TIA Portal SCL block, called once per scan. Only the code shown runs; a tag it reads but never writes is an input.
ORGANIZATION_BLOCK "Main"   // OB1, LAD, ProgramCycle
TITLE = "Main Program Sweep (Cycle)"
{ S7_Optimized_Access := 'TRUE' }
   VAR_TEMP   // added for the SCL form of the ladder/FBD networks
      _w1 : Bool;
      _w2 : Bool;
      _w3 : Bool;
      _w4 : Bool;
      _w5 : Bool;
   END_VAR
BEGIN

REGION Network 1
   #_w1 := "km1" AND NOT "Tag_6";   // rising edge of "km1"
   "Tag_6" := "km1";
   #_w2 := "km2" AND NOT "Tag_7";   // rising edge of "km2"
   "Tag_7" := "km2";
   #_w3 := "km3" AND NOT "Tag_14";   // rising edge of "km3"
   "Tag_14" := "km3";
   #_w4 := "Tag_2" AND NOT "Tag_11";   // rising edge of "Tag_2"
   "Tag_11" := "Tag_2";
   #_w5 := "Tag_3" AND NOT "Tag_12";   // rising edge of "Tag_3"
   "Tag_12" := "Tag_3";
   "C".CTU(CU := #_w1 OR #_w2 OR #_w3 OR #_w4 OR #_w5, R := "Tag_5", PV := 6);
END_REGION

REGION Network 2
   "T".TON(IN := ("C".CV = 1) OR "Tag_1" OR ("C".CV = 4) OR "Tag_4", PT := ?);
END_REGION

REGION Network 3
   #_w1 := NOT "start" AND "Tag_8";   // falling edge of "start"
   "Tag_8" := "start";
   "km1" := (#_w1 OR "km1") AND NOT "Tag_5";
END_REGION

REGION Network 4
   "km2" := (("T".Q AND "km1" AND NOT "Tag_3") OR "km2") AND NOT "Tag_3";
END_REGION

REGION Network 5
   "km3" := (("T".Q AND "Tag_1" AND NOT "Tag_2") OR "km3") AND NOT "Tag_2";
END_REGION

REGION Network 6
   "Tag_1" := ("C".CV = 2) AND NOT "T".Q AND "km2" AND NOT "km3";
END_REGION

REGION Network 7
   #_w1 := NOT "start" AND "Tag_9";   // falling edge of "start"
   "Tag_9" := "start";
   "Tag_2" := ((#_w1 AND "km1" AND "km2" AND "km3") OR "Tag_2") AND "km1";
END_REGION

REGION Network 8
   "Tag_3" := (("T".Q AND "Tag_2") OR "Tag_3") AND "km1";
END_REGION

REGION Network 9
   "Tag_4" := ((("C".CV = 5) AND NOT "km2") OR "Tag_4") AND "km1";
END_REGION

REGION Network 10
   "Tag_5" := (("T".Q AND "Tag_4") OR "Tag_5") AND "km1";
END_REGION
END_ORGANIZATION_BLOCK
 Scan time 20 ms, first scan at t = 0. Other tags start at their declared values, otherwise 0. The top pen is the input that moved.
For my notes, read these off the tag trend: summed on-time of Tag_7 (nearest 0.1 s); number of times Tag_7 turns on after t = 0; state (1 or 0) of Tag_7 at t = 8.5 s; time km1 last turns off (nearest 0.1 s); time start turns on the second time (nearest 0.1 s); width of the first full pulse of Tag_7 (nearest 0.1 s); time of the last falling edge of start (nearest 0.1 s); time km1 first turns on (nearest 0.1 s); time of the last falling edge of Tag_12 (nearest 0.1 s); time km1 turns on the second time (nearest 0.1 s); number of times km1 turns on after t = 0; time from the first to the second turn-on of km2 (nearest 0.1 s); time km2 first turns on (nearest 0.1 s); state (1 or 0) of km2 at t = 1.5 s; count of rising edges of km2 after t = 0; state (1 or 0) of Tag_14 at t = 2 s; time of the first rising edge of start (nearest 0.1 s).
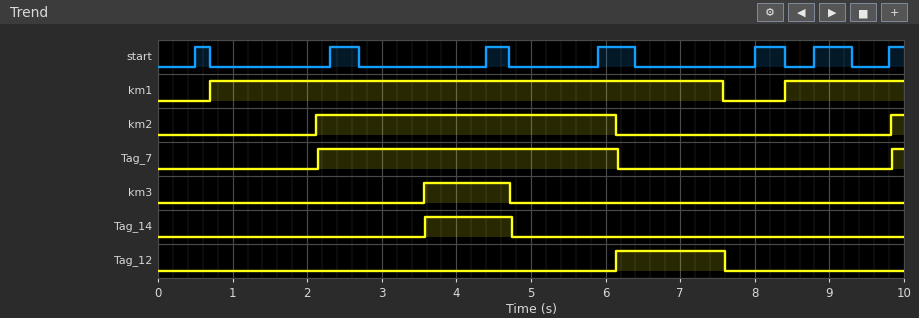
4.2 s
2
0
7.6 s
2.3 s
4.0 s
9.3 s
0.7 s
7.6 s
8.4 s
2
7.7 s
2.1 s
0
2
0
0.5 s
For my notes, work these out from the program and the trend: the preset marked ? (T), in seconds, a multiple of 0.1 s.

1.4 s
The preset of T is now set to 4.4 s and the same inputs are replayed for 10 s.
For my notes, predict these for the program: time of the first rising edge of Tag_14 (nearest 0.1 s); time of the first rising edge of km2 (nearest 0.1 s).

9.6 s
5.1 s
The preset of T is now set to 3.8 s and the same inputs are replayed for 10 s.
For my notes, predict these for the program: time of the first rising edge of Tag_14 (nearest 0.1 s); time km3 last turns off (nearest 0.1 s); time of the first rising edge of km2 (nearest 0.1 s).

8.4 s
8.4 s
4.5 s
